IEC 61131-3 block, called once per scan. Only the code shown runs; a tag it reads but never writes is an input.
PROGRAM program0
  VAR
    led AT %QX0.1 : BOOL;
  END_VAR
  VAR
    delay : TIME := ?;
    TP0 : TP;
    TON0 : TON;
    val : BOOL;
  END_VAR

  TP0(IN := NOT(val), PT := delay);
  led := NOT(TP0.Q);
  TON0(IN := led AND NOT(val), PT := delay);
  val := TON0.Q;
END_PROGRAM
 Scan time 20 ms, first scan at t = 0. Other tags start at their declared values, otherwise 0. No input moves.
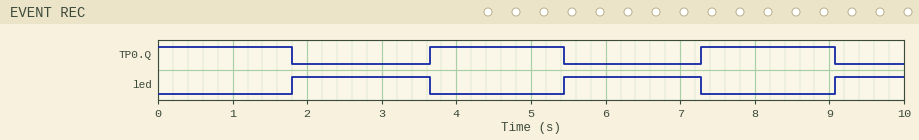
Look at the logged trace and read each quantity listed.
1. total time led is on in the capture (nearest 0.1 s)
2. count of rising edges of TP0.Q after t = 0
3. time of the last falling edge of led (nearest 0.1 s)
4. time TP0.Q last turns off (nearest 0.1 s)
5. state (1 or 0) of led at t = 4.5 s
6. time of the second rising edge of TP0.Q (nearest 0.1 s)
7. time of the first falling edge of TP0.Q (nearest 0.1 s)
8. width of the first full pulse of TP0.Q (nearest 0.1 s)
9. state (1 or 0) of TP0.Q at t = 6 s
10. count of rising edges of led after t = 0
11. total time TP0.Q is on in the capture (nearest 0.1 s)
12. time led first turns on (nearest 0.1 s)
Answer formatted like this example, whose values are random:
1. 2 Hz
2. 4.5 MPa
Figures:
1. 4.6 s
2. 2
3. 7.3 s
4. 9.1 s
5. 0
6. 7.3 s
7. 1.8 s
8. 1.8 s
9. 0
10. 3
11. 5.4 s
12. 1.8 s
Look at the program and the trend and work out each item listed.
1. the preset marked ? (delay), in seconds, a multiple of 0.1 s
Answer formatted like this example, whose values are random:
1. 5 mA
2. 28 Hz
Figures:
1. 1.8 s
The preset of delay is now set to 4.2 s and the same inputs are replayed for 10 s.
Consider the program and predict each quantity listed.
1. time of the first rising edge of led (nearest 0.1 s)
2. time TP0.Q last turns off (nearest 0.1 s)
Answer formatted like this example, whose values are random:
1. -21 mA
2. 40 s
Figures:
1. 4.2 s
2. 4.2 s
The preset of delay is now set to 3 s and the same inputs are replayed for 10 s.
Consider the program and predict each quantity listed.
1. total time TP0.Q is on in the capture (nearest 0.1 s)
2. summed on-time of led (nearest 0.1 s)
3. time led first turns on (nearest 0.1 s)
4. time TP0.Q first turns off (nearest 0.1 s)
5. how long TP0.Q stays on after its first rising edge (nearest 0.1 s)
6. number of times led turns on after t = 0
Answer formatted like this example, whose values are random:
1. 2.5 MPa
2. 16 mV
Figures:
1. 6.0 s
2. 4.0 s
3. 3.0 s
4. 3.0 s
5. 3.0 s
6. 2
